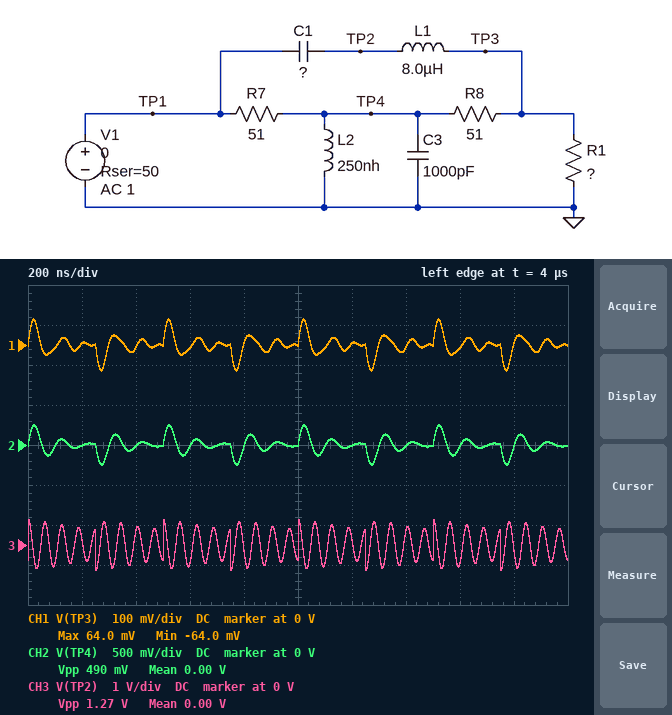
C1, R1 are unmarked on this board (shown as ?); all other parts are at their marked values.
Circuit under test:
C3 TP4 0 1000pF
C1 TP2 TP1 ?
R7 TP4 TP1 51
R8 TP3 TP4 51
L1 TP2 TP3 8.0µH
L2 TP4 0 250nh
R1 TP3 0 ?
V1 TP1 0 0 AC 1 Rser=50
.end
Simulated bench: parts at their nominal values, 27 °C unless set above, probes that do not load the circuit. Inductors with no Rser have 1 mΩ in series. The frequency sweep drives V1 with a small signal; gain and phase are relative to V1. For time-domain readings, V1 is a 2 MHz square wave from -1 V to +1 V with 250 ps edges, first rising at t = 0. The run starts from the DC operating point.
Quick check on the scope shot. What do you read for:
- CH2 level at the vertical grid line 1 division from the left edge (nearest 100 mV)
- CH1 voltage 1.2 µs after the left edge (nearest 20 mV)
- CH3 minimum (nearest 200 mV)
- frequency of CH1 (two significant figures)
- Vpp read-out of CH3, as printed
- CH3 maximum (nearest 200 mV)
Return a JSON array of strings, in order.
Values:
["0 V", "0 V", "-600 mV", "2.0 MHz", "1.27 V", "600 mV"]
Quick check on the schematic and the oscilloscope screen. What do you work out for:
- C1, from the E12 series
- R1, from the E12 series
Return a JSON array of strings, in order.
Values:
["12 pF", "15 Ω"]
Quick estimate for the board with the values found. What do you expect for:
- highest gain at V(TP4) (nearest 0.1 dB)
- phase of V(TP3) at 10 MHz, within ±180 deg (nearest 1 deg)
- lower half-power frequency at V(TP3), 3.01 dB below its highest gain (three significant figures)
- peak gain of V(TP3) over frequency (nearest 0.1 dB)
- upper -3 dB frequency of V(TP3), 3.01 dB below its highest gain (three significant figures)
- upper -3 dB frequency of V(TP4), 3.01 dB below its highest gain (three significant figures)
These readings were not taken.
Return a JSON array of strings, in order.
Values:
["-8.1 dB", "6 deg", "16.0 MHz", "-15.1 dB", "16.8 MHz", "12.2 MHz"]
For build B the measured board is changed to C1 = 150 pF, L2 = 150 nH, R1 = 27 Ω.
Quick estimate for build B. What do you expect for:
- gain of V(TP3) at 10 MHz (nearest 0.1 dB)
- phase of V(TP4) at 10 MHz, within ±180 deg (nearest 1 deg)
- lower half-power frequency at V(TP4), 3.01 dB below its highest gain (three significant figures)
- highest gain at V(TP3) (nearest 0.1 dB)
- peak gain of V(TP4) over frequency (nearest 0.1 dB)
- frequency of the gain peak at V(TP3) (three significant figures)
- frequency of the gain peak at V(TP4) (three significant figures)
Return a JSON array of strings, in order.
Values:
["-25.5 dB", "63 deg", "11.3 MHz", "-13.5 dB", "-7.2 dB", "4.56 MHz", "13.0 MHz"]
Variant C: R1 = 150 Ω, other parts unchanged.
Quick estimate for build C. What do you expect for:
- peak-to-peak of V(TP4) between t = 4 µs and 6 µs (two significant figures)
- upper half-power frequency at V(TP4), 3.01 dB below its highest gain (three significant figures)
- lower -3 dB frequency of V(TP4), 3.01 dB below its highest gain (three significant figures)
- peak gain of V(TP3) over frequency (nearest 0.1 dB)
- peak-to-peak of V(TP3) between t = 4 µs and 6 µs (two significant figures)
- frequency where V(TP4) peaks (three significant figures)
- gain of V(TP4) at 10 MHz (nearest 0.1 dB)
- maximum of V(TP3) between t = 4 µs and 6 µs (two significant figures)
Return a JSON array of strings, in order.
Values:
["630 mV", "11.3 MHz", "8.95 MHz", "-6.0 dB", "520 mV", "10.1 MHz", "-3.5 dB", "260 mV"]
